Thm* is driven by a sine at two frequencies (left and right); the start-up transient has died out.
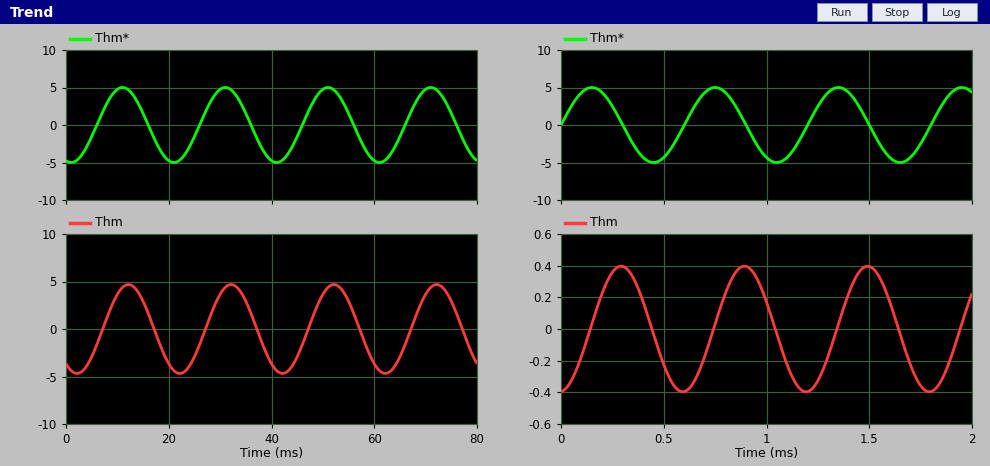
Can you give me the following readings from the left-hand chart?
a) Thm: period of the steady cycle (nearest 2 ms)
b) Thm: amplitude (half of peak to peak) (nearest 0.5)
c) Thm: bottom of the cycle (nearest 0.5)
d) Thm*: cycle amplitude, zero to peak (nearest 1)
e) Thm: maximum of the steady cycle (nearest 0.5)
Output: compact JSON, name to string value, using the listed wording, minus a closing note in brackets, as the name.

{"Thm: period of the steady cycle": "20 ms", "Thm: amplitude (half of peak to peak)": "4.5", "Thm: bottom of the cycle": "-4.5", "Thm*: cycle amplitude, zero to peak": "5", "Thm: maximum of the steady cycle": "4.5"}
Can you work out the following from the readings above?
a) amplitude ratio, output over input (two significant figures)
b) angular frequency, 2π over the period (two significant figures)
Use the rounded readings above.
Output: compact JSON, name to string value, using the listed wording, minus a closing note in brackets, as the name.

{"amplitude ratio, output over input": "0.90", "angular frequency, 2π over the period": "0.31 rad/ms"}
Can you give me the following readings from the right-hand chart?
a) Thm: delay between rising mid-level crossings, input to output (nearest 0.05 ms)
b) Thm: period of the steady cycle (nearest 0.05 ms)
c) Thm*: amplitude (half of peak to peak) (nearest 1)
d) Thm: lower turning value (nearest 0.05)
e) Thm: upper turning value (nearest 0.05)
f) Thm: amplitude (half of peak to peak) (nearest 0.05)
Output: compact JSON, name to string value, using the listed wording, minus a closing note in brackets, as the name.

{"Thm: delay between rising mid-level crossings, input to output": "0.15 ms", "Thm: period of the steady cycle": "0.60 ms", "Thm*: amplitude (half of peak to peak)": "5", "Thm: lower turning value": "-0.40", "Thm: upper turning value": "0.40", "Thm: amplitude (half of peak to peak)": "0.40"}
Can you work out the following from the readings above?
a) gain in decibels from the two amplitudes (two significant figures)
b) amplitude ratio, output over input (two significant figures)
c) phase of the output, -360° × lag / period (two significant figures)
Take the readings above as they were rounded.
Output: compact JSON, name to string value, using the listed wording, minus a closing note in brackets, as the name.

{"gain in decibels from the two amplitudes": "-22 dB", "amplitude ratio, output over input": "0.080", "phase of the output, -360° × lag / period": "-90°"}
